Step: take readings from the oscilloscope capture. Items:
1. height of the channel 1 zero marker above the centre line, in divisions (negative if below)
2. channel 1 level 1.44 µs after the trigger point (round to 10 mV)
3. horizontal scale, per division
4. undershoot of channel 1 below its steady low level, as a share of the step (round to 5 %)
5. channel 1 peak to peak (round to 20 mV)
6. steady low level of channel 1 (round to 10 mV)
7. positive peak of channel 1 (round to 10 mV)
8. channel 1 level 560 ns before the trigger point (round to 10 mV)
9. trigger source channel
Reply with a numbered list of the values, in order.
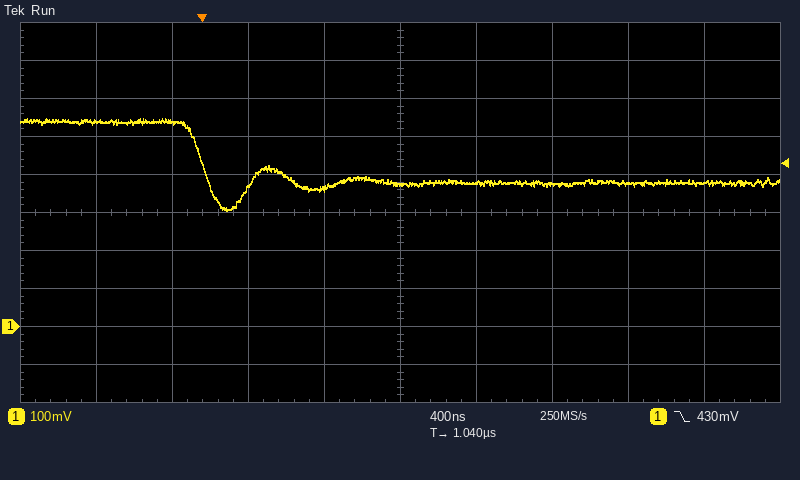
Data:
1. -3.0 div
2. 380 mV
3. 400 ns
4. 45 %
5. 240 mV
6. 380 mV
7. 550 mV
8. 540 mV
9. channel 1
